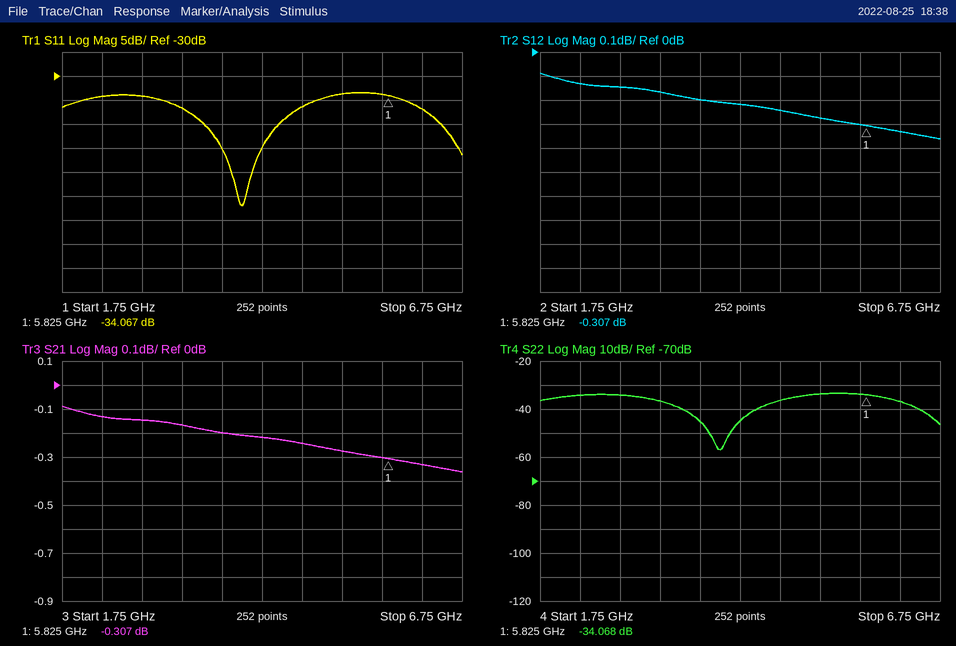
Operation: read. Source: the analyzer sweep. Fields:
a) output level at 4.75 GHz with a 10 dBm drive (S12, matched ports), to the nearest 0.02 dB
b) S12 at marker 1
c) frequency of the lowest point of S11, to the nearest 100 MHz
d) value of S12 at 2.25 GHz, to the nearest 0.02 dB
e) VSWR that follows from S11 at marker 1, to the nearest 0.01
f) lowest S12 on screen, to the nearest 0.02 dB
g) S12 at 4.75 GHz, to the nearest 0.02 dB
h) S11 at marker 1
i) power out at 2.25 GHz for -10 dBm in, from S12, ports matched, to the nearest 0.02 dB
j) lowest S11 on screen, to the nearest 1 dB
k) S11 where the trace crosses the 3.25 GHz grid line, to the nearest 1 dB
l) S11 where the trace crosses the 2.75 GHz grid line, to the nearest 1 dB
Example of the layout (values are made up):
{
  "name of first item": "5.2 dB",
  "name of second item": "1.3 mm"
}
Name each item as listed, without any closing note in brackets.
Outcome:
{
  "output level at 4.75 GHz with a 10 dBm drive (S12, matched ports), to the nearest 0.02 dB": "9.76 dBm",
  "S12 at marker 1": "-0.307 dB",
  "frequency of the lowest point of S11, to the nearest 100 MHz": "4.0 GHz",
  "value of S12 at 2.25 GHz, to the nearest 0.02 dB": "-0.14 dB",
  "VSWR that follows from S11 at marker 1, to the nearest 0.01": "1.04",
  "lowest S12 on screen, to the nearest 0.02 dB": "-0.36 dB",
  "S12 at 4.75 GHz, to the nearest 0.02 dB": "-0.24 dB",
  "S11 at marker 1": "-34.067 dB",
  "power out at 2.25 GHz for -10 dBm in, from S12, ports matched, to the nearest 0.02 dB": "-10.14 dBm",
  "lowest S11 on screen, to the nearest 1 dB": "-57 dB",
  "S11 where the trace crosses the 3.25 GHz grid line, to the nearest 1 dB": "-37 dB",
  "S11 where the trace crosses the 2.75 GHz grid line, to the nearest 1 dB": "-34 dB"
}
